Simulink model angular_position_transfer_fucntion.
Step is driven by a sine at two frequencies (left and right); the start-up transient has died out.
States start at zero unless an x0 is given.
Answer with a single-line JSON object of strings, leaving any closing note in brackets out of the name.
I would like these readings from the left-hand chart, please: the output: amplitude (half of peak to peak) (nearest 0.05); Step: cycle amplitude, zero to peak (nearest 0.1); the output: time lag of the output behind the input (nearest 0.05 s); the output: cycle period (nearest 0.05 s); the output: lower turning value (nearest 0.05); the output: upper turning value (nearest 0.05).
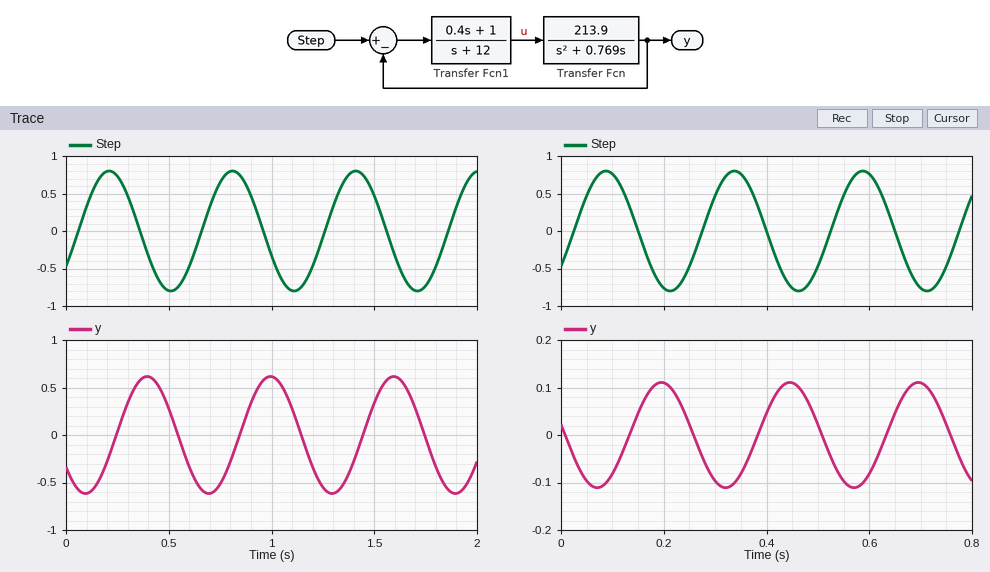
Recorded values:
{"the output: amplitude (half of peak to peak)": "0.60", "Step: cycle amplitude, zero to peak": "0.8", "the output: time lag of the output behind the input": "0.20 s", "the output: cycle period": "0.60 s", "the output: lower turning value": "-0.60", "the output: upper turning value": "0.60"}
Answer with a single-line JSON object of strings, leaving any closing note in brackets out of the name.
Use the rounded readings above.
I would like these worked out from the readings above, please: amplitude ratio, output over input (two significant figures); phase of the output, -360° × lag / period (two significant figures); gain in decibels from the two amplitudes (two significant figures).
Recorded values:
{"amplitude ratio, output over input": "0.75", "phase of the output, -360° × lag / period": "-120°", "gain in decibels from the two amplitudes": "-2.5 dB"}
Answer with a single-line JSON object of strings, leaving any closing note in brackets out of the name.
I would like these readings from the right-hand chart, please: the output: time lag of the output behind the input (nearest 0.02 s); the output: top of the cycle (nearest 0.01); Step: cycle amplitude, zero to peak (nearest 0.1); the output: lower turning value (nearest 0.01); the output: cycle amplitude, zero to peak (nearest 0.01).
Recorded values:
{"the output: time lag of the output behind the input": "0.10 s", "the output: top of the cycle": "0.11", "Step: cycle amplitude, zero to peak": "0.8", "the output: lower turning value": "-0.11", "the output: cycle amplitude, zero to peak": "0.11"}
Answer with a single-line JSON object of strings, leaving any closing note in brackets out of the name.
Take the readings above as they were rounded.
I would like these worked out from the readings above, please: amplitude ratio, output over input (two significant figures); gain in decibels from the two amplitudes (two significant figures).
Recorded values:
{"amplitude ratio, output over input": "0.14", "gain in decibels from the two amplitudes": "-17 dB"}
